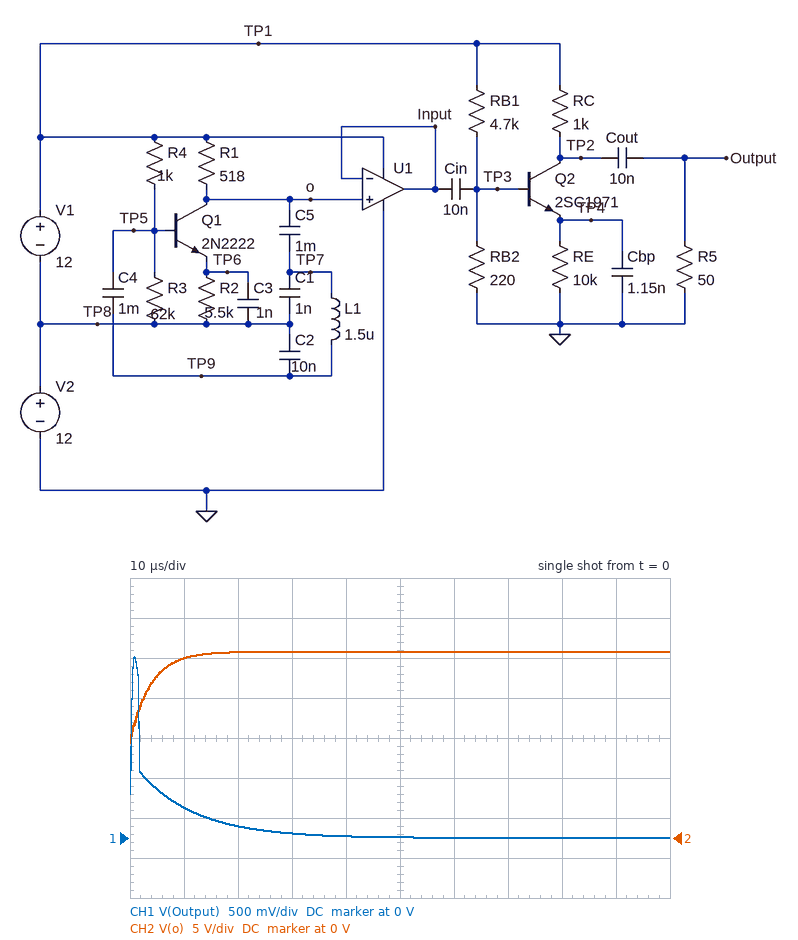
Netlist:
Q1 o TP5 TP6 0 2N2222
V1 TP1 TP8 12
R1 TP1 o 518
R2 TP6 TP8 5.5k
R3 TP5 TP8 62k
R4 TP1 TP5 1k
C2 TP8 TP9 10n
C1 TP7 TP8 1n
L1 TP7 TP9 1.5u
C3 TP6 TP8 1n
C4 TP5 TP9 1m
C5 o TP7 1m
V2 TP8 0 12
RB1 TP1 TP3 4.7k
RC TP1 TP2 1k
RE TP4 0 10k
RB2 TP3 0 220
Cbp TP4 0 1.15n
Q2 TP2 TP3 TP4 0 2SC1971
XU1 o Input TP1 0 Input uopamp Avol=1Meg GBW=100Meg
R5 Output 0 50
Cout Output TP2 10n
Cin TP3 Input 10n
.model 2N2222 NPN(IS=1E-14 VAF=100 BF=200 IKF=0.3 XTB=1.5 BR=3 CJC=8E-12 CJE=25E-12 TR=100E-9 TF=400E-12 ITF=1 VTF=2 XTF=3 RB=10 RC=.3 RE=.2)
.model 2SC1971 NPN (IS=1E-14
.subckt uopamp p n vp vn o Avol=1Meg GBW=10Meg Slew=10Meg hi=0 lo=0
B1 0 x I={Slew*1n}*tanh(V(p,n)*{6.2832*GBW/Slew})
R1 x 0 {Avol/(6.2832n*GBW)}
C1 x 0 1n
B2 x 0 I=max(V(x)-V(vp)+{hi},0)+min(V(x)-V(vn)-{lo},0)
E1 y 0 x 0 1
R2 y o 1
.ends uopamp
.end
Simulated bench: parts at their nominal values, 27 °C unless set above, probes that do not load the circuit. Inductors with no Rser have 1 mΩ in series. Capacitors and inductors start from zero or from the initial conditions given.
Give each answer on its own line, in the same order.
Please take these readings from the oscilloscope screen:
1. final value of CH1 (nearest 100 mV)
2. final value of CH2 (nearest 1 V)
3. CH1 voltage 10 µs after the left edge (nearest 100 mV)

0 V
23 V
400 mV
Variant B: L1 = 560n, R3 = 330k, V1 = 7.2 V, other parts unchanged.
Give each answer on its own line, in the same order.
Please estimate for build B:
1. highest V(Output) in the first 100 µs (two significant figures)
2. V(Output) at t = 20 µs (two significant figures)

2.2 V
110 mV
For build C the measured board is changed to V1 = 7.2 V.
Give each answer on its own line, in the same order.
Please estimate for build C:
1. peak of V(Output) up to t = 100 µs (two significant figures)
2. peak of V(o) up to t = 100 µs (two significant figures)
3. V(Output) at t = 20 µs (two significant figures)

2.2 V
19 V
110 mV
